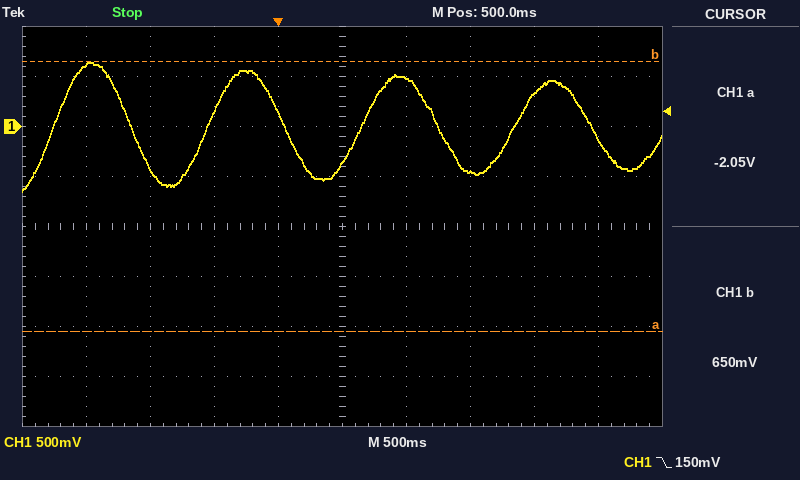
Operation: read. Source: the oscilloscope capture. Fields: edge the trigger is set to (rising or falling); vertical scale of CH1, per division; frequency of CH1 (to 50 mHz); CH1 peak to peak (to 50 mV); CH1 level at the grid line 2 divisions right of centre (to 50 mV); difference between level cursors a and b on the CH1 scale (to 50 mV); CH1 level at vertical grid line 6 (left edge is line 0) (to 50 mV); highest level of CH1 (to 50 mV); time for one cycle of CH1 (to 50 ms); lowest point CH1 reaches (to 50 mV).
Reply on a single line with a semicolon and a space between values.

falling; 500 mV; 850 mHz; 1.30 V; -450 mV; 2.70 V; 500 mV; 650 mV; 1.20 s; -650 mV
